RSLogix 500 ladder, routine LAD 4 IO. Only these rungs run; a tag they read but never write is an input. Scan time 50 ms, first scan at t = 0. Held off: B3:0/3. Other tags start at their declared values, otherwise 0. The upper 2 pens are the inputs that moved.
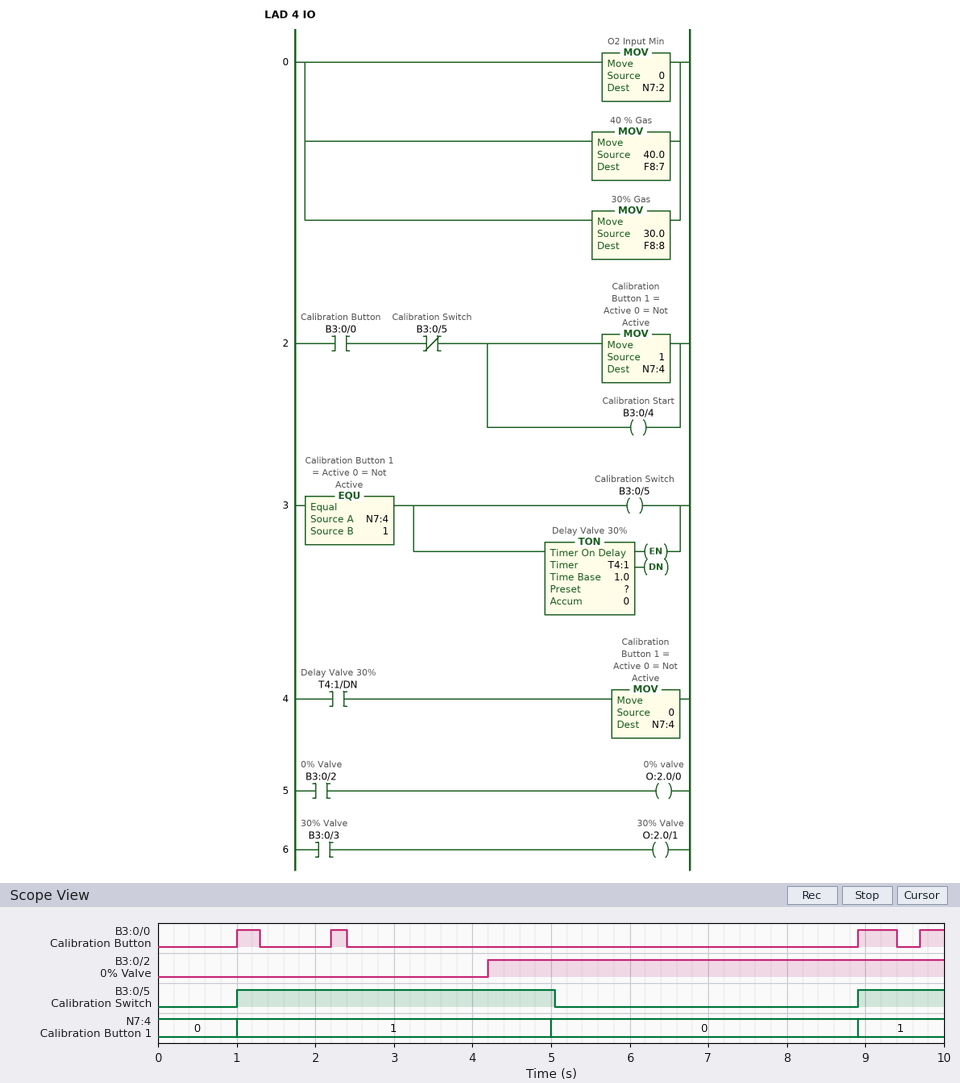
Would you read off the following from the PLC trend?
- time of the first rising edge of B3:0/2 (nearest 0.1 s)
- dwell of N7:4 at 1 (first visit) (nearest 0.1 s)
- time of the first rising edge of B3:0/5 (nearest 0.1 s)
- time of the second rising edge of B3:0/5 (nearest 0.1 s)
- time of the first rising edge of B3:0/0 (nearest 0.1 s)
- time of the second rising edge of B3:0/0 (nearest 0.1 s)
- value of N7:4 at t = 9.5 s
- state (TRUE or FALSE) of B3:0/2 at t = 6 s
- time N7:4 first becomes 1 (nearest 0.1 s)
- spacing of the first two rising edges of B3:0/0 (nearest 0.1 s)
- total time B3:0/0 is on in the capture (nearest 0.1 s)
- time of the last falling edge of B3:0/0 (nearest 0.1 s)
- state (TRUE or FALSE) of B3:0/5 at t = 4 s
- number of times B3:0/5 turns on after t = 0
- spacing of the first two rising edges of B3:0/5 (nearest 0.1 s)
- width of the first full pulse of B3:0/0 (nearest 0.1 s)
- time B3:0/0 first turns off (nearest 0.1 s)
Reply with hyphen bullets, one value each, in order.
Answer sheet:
- 4.2 s
- 4.0 s
- 1.0 s
- 8.9 s
- 1.0 s
- 2.2 s
- 1
- TRUE
- 1.0 s
- 1.2 s
- 1.3 s
- 9.4 s
- TRUE
- 2
- 7.9 s
- 0.3 s
- 1.3 s
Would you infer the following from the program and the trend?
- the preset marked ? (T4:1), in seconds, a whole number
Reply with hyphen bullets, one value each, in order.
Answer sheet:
- 4 s
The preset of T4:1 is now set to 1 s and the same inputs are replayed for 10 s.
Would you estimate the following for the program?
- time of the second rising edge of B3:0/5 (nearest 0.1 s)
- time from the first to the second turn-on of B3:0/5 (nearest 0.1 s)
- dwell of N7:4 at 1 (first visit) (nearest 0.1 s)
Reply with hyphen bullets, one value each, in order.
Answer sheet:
- 2.2 s
- 1.2 s
- 1.0 s
